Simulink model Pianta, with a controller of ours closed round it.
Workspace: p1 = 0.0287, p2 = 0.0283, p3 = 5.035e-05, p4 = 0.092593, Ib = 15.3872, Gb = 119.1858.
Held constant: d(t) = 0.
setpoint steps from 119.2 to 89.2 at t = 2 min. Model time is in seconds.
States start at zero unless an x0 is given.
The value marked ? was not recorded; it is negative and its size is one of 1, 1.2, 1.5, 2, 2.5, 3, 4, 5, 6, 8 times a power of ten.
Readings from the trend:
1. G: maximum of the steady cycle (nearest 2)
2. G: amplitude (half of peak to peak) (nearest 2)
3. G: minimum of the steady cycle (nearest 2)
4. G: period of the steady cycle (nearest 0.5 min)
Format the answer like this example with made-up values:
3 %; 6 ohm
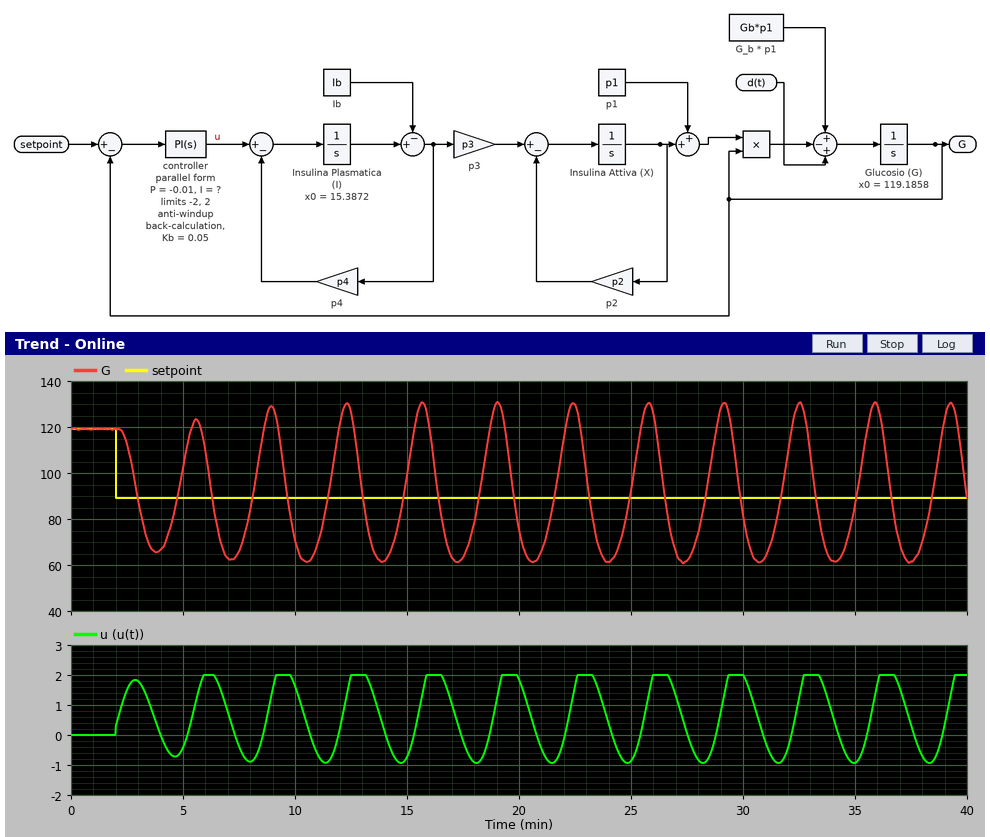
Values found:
130; 34; 62; 3.5 min
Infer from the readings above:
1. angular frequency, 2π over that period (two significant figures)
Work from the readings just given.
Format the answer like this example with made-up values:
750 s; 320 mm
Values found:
1.8 rad/min
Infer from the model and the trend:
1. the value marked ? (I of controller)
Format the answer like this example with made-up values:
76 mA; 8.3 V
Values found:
-0.0015
